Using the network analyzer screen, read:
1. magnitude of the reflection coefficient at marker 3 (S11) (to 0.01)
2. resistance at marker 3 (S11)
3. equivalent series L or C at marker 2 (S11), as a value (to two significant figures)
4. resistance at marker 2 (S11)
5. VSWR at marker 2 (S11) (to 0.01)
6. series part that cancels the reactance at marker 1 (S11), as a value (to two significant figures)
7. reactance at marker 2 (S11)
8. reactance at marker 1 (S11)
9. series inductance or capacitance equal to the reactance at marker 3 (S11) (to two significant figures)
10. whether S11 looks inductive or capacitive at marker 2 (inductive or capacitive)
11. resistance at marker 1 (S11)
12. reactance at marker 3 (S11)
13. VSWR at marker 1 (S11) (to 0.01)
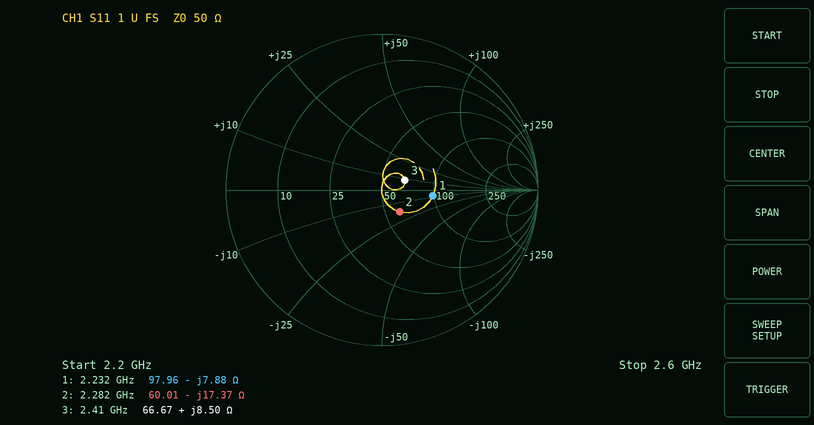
0.16
66.67 Ω
4.0 pF
60.01 Ω
1.44
560 pH
-17.37 Ω
-7.88 Ω
560 pH
capacitive
97.96 Ω
+8.50 Ω
1.98
